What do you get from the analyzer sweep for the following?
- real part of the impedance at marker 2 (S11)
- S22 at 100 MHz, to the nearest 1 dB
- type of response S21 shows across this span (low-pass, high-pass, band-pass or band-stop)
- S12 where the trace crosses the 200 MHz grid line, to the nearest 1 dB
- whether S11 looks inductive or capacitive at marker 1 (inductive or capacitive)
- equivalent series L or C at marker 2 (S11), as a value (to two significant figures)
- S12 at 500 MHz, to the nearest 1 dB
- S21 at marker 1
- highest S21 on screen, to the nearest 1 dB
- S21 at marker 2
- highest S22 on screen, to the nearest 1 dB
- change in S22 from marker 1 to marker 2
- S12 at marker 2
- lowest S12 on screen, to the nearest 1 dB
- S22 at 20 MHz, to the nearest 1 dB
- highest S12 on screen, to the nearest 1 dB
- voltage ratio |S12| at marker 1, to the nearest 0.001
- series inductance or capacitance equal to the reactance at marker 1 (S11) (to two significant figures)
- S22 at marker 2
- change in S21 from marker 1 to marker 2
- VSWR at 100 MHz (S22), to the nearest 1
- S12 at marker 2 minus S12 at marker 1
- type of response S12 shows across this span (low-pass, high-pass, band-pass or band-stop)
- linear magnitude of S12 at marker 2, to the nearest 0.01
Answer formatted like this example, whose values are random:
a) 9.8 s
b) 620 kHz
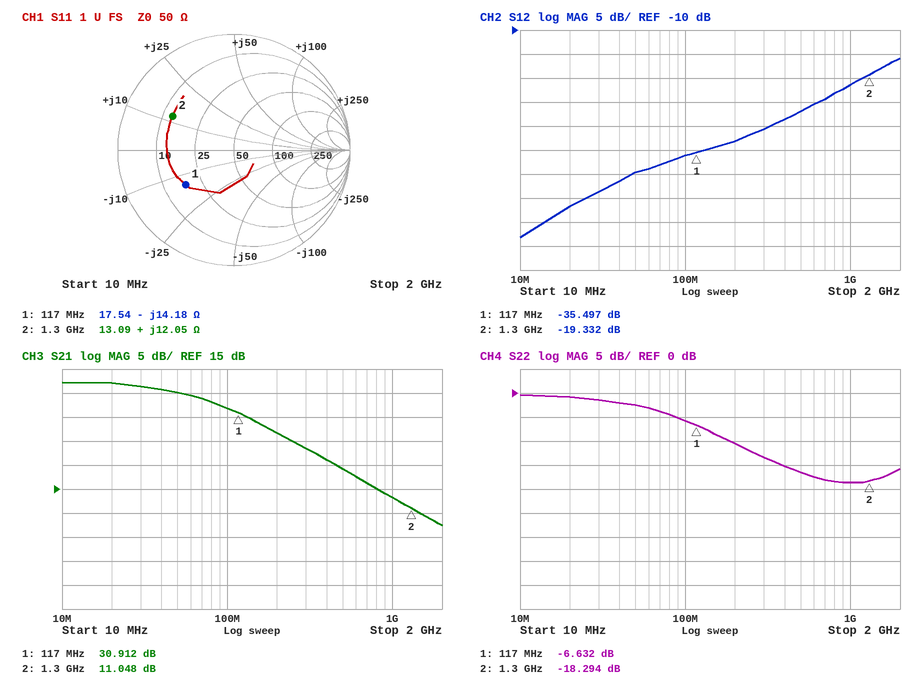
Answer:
a) 13.09 Ω
b) -6 dB
c) low-pass
d) -33 dB
e) capacitive
f) 1.5 nH
g) -27 dB
h) 30.912 dB
i) 37 dB
j) 11.048 dB
k) 0 dB
l) -11.662 dB
m) -19.332 dB
n) -53 dB
o) -1 dB
p) -16 dB
q) 0.017
r) 96 pF
s) -18.294 dB
t) -19.864 dB
u) 3
v) 16.165 dB
w) high-pass
x) 0.11
